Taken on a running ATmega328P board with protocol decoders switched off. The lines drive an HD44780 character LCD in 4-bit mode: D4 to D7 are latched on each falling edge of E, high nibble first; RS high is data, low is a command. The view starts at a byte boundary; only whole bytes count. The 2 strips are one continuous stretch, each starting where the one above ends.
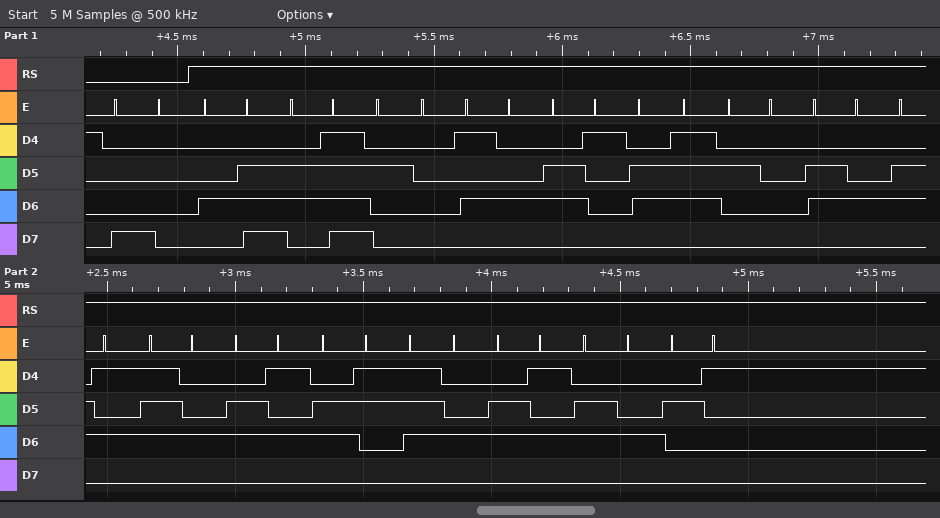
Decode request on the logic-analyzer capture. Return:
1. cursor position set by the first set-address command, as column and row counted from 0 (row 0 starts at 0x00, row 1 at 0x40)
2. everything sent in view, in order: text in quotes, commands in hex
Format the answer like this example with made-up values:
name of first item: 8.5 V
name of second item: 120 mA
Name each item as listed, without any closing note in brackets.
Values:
cursor position set by the first set-address command, as column and row counted from 0: column 0, row 0
everything sent in view, in order: text in quotes, commands in hex: 0x80 "No Tag detected!"
